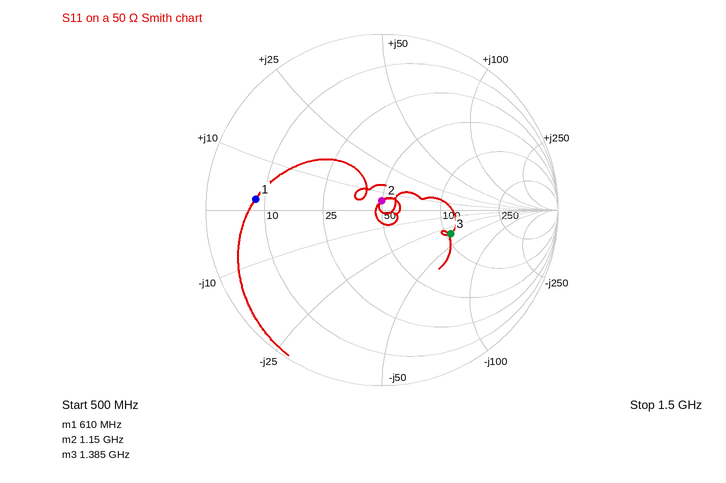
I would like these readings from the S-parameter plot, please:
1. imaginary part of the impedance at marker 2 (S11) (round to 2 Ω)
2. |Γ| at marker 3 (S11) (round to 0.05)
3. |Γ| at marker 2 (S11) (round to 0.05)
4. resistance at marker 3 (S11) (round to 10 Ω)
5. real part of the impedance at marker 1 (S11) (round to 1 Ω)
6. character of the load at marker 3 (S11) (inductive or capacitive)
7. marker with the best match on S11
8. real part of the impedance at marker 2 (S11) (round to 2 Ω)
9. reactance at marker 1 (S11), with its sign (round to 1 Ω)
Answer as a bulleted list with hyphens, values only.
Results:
- +6 Ω
- 0.40
- 0.05
- 110 Ω
- 8 Ω
- capacitive
- marker 2
- 50 Ω
- +2 Ω
